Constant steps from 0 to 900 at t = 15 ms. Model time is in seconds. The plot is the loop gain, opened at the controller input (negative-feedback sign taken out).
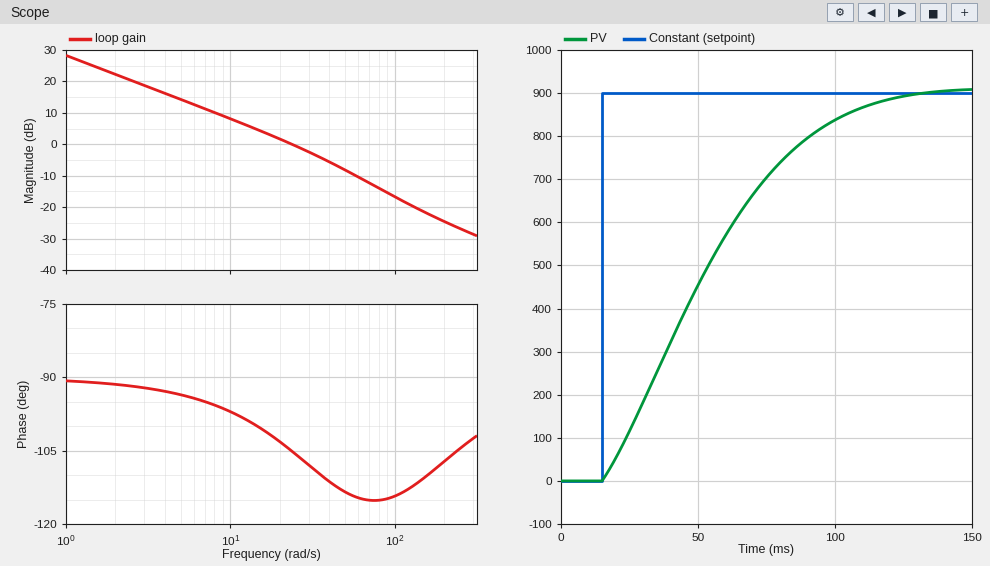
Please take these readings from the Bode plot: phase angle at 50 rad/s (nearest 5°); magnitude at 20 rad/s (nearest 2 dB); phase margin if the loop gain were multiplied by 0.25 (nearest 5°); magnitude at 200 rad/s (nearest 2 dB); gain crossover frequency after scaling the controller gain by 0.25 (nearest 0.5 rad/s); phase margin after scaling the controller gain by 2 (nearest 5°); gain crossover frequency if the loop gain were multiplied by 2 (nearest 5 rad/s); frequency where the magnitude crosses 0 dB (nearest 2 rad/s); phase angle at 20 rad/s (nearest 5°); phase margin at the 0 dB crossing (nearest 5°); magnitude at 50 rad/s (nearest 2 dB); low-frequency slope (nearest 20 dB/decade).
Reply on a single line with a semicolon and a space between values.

-115°; 2 dB; 85°; -24 dB; 6.5 rad/s; 70°; 40 rad/s; 24 rad/s; -105°; 75°; -8 dB; -20 dB/decade
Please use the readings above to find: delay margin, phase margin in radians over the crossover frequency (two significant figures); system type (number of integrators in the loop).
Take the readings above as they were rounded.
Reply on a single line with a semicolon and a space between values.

0.055 s; 1
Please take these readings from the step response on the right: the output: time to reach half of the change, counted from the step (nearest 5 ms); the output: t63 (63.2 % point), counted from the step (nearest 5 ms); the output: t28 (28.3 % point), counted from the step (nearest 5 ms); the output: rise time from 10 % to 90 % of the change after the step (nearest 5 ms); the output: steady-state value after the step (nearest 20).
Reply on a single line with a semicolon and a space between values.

35 ms; 45 ms; 20 ms; 70 ms; 900
